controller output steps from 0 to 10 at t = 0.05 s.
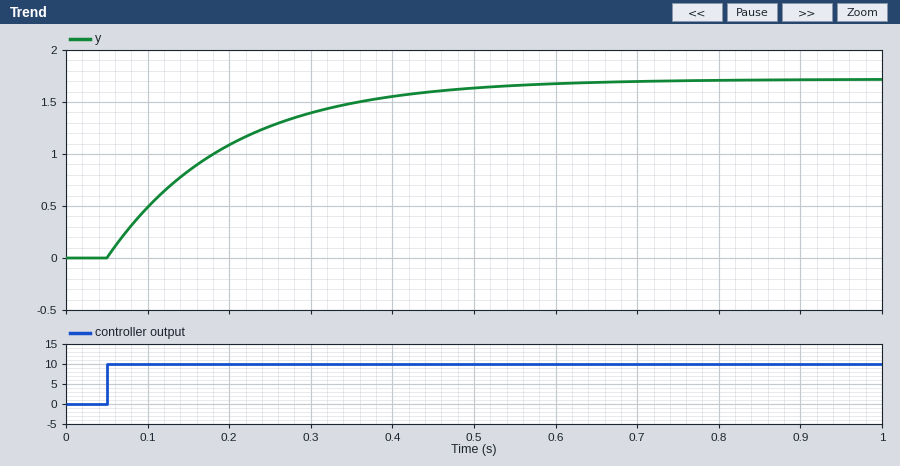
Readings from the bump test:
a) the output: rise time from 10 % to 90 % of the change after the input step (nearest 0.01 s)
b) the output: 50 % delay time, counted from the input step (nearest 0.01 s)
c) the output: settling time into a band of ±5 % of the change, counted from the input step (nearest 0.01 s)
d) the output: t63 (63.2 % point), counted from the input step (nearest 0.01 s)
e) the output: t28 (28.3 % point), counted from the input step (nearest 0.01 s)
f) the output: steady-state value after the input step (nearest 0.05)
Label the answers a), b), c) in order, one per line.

a) 0.33 s
b) 0.10 s
c) 0.45 s
d) 0.15 s
e) 0.05 s
f) 1.70
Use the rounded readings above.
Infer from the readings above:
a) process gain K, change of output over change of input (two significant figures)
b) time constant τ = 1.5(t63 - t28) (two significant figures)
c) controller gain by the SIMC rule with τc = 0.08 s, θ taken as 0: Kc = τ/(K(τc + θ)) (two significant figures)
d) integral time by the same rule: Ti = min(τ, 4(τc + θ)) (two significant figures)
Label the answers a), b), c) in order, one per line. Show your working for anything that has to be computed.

a) (1.7 - 0) / 10 = 0.17
b) 1.5 × (0.15 - 0.05) = 0.15 s
c) 0.15 / (0.17 × (0.08 + 0)) = 11
d) min(0.15, 4 × (0.08 + 0)) = 0.15 s
